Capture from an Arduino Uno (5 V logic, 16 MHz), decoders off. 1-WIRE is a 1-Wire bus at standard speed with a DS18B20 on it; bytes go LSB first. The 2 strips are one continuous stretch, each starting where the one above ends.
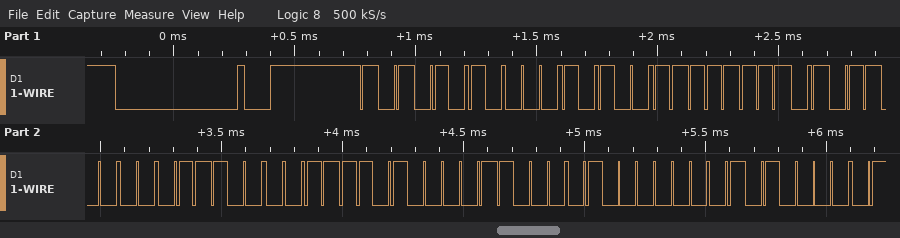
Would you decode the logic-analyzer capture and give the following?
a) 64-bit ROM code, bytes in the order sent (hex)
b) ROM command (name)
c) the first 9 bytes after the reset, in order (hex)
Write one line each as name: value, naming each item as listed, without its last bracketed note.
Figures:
64-bit ROM code, bytes in the order sent: 28 FF 1A 1C 5E 18 02 0A
ROM command: Match ROM
the first 9 bytes after the reset, in order: 55 28 FF 1A 1C 5E 18 02 0A
